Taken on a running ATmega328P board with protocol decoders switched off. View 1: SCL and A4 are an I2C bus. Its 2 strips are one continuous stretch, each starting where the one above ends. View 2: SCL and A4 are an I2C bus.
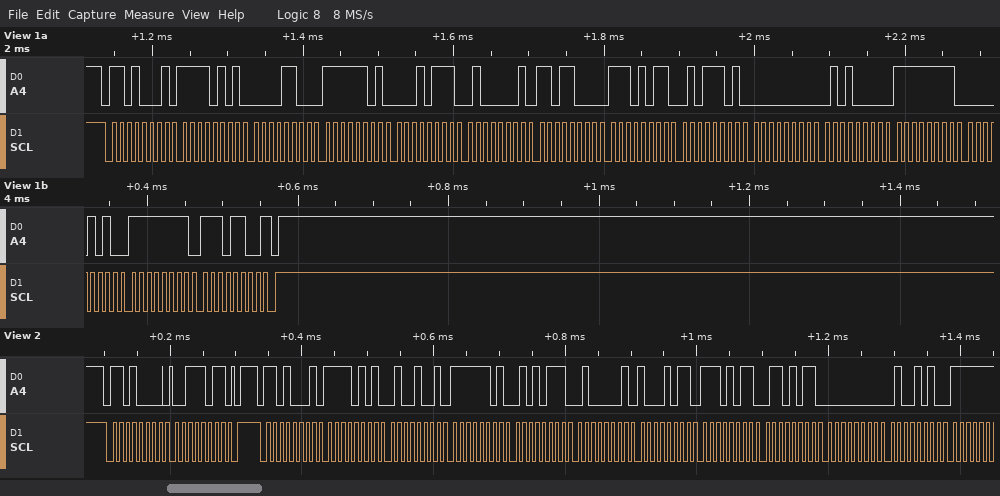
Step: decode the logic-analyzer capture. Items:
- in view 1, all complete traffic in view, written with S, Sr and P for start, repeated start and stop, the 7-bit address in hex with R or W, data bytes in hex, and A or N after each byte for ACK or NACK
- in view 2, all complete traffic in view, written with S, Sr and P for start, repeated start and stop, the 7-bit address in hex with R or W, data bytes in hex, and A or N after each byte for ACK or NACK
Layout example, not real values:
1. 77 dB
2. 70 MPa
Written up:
1. S 68R A F5 A 0C A FD A 17 A 41 A D8 A EB A 5D A 00 A 50 A FF A 0A A FF A EC N P
2. S 68W A 3B A P S 68R A F5 A 49 A FD A 57 A 41 A 8B A EB A 6B A 00 A 4A A
